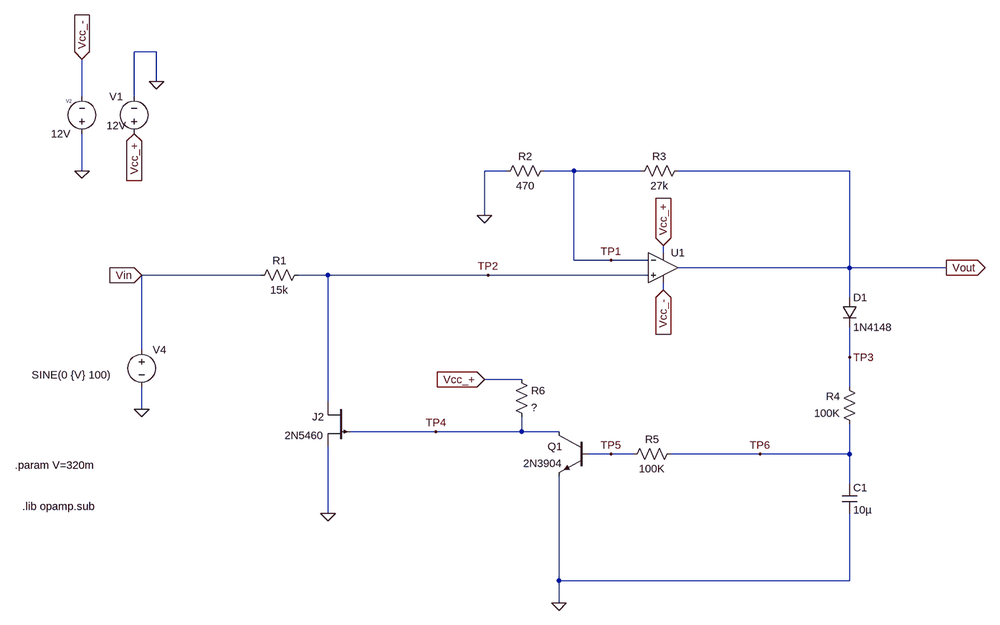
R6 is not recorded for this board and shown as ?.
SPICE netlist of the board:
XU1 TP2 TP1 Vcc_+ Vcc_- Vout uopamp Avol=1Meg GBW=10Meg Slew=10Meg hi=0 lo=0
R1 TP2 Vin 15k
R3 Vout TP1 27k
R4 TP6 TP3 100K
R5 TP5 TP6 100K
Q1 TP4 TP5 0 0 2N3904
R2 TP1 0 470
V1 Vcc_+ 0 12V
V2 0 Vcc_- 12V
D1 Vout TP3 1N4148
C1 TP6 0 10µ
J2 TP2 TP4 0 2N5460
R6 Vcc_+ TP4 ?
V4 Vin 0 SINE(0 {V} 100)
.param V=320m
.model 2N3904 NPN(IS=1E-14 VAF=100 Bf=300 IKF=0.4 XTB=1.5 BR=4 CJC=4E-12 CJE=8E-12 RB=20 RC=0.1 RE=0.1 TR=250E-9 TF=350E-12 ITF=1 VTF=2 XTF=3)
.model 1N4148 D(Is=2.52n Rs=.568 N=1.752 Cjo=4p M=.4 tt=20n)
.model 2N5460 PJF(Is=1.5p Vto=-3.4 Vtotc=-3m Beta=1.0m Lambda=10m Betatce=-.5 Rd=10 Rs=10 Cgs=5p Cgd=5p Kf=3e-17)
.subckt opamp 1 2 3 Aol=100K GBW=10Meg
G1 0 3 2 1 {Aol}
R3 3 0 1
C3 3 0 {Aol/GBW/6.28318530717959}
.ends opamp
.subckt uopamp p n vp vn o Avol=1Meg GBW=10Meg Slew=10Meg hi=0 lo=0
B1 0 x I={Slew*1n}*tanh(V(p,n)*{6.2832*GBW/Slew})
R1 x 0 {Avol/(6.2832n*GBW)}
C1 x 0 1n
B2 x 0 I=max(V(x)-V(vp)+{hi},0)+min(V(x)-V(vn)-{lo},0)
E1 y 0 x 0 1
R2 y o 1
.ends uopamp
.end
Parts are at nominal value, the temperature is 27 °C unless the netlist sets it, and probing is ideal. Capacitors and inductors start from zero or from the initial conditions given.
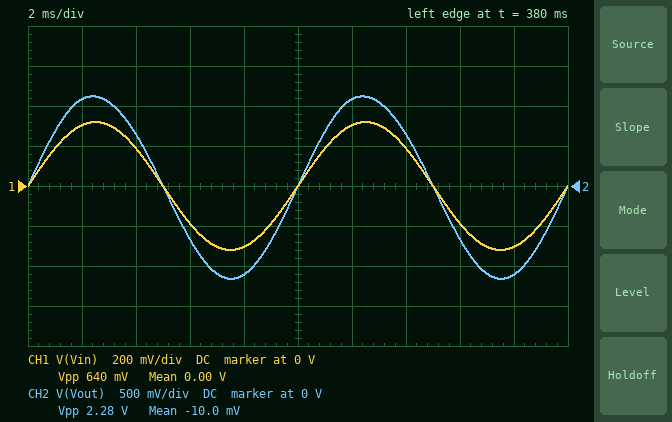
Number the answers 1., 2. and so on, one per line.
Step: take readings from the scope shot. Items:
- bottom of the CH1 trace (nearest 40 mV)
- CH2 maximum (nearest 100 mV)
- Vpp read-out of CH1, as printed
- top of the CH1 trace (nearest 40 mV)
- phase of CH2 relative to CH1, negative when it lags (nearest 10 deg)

1. -320 mV
2. 1.1 V
3. 640 mV
4. 320 mV
5. 0 deg
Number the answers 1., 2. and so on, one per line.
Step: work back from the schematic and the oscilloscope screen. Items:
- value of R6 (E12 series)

1. 100 kΩ
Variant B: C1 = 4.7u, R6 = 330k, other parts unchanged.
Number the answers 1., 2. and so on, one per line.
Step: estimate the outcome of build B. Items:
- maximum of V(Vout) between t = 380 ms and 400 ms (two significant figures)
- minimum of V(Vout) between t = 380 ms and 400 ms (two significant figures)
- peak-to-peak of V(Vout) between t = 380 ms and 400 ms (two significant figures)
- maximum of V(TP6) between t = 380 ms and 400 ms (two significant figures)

1. 900 mV
2. -920 mV
3. 1.8 V
4. 570 mV
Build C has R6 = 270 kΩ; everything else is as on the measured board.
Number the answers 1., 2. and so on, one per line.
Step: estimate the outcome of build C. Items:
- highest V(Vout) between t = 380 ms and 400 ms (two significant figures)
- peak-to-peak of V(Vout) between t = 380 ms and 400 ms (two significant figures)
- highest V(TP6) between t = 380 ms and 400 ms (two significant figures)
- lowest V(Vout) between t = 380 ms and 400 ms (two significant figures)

1. 930 mV
2. 1.9 V
3. 580 mV
4. -950 mV
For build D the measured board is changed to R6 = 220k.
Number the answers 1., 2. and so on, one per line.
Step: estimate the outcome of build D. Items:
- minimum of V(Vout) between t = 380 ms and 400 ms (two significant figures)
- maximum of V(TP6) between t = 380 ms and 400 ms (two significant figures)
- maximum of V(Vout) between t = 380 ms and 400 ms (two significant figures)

1. -990 mV
2. 590 mV
3. 960 mV
